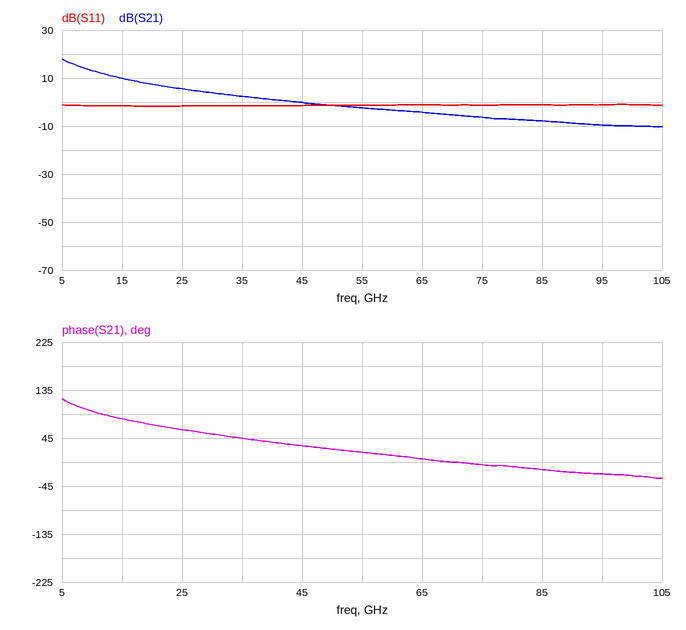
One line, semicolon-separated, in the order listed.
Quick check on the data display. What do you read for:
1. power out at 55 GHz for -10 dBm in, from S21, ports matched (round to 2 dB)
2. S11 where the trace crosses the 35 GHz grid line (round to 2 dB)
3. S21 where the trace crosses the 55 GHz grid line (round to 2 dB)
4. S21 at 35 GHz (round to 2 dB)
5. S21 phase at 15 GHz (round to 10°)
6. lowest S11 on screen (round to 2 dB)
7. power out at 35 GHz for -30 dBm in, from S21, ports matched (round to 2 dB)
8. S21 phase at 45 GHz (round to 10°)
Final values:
-12 dBm; -2 dB; -2 dB; 2 dB; 80°; -2 dB; -28 dBm; 30°
